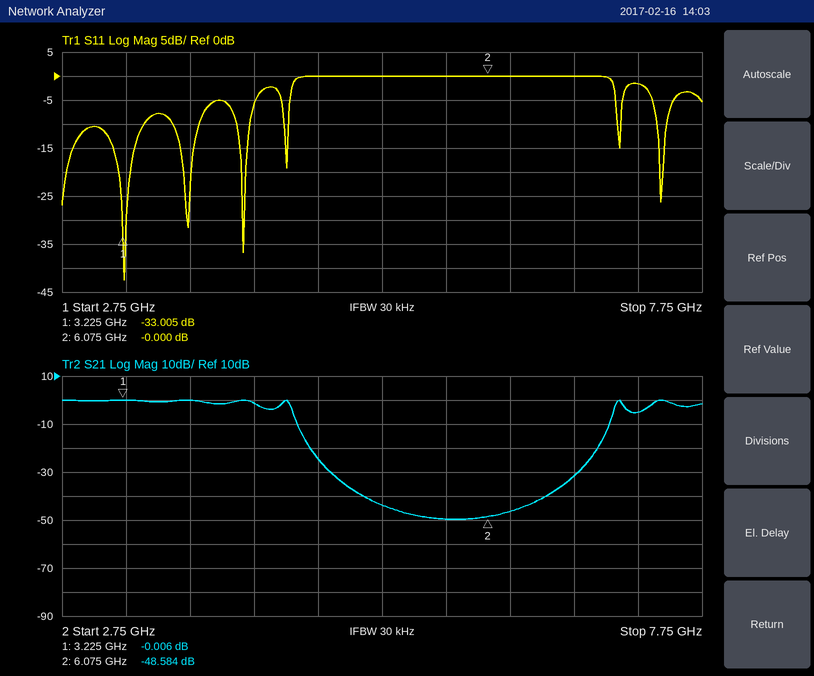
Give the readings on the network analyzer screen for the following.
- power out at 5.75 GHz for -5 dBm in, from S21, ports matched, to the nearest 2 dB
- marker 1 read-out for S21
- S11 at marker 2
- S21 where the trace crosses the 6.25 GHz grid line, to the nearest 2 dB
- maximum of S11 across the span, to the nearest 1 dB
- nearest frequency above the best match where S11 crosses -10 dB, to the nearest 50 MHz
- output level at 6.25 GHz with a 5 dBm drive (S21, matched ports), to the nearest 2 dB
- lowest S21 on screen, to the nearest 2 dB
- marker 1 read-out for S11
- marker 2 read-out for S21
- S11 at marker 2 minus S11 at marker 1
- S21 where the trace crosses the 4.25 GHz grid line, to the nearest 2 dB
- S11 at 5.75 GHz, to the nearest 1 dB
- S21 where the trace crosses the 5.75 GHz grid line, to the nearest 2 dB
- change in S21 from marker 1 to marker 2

-54 dBm
-0.006 dB
-0.000 dB
-46 dB
0 dB
3.40 GHz
-42 dBm
-50 dB
-33.005 dB
-48.584 dB
33.005 dB
-2 dB
0 dB
-50 dB
-48.578 dB
